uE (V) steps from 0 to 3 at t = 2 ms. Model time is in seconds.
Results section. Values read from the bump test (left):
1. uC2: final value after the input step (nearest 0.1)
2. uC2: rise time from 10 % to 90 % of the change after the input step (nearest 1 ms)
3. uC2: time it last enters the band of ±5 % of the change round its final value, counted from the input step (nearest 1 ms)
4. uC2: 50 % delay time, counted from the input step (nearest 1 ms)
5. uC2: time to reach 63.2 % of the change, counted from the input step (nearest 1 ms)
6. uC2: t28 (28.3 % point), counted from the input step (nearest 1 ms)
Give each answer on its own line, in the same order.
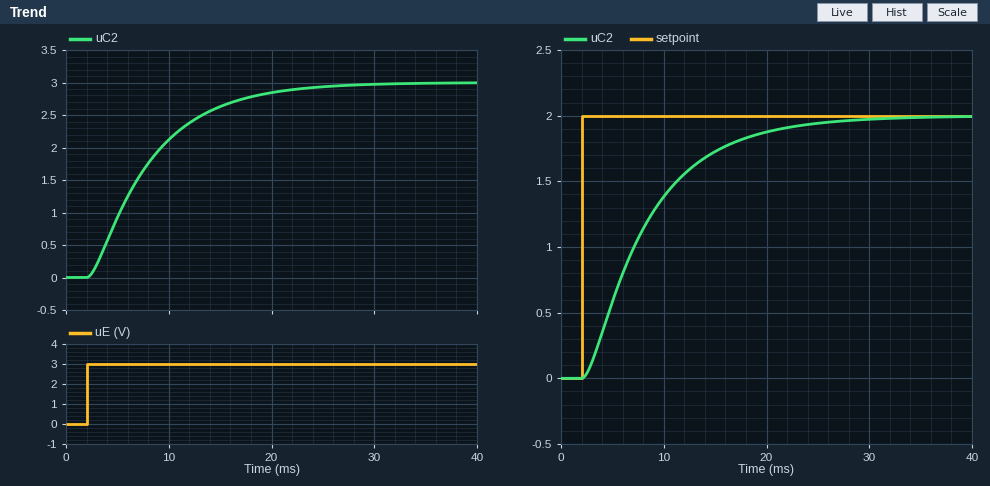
3.0
13 ms
18 ms
5 ms
7 ms
3 ms
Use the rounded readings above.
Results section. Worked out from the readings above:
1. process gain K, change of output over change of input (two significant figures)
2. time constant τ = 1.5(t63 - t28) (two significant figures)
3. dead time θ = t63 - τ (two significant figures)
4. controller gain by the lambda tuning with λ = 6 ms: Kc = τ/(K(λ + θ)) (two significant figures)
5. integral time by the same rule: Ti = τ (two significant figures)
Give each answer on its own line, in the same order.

1.0
6.0 ms
1.0 ms
0.86
6.0 ms
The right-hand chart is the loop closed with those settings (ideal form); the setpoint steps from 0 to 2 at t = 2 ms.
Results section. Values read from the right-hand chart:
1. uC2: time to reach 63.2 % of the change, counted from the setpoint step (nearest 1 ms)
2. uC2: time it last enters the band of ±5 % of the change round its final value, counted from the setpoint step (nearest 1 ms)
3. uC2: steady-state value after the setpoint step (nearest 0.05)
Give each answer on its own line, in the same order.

7 ms
19 ms
2.00
